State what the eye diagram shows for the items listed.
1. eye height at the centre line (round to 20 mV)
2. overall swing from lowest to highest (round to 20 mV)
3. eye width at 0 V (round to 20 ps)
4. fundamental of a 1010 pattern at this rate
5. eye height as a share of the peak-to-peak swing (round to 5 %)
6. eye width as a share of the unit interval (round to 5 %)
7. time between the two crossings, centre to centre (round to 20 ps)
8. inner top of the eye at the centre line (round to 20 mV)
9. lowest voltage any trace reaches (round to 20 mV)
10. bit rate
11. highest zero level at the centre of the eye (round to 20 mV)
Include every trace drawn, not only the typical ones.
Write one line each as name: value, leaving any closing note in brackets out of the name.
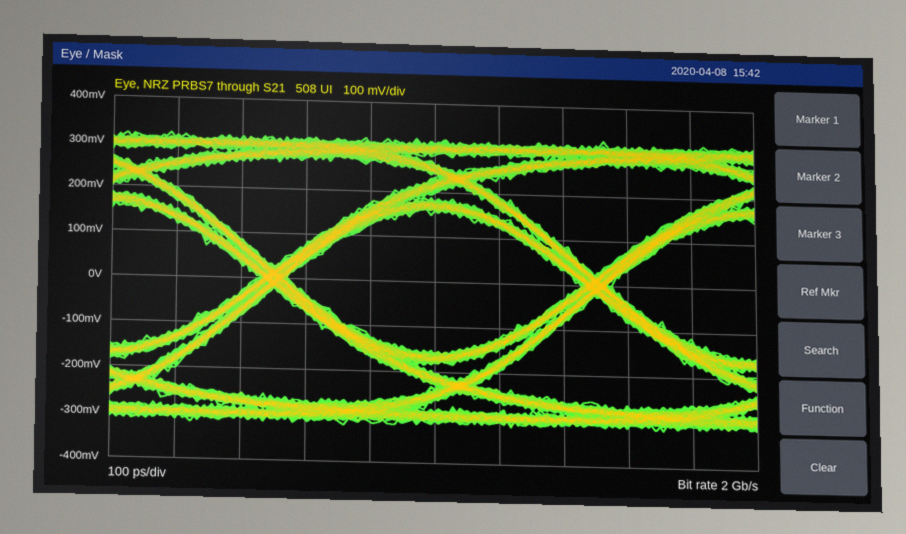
eye height at the centre line: 320 mV
overall swing from lowest to highest: 640 mV
eye width at 0 V: 460 ps
fundamental of a 1010 pattern at this rate: 1 GHz
eye height as a share of the peak-to-peak swing: 50 %
eye width as a share of the unit interval: 90 %
time between the two crossings, centre to centre: 500 ps
inner top of the eye at the centre line: 160 mV
lowest voltage any trace reaches: -320 mV
bit rate: 2 Gb/s
highest zero level at the centre of the eye: -160 mV
